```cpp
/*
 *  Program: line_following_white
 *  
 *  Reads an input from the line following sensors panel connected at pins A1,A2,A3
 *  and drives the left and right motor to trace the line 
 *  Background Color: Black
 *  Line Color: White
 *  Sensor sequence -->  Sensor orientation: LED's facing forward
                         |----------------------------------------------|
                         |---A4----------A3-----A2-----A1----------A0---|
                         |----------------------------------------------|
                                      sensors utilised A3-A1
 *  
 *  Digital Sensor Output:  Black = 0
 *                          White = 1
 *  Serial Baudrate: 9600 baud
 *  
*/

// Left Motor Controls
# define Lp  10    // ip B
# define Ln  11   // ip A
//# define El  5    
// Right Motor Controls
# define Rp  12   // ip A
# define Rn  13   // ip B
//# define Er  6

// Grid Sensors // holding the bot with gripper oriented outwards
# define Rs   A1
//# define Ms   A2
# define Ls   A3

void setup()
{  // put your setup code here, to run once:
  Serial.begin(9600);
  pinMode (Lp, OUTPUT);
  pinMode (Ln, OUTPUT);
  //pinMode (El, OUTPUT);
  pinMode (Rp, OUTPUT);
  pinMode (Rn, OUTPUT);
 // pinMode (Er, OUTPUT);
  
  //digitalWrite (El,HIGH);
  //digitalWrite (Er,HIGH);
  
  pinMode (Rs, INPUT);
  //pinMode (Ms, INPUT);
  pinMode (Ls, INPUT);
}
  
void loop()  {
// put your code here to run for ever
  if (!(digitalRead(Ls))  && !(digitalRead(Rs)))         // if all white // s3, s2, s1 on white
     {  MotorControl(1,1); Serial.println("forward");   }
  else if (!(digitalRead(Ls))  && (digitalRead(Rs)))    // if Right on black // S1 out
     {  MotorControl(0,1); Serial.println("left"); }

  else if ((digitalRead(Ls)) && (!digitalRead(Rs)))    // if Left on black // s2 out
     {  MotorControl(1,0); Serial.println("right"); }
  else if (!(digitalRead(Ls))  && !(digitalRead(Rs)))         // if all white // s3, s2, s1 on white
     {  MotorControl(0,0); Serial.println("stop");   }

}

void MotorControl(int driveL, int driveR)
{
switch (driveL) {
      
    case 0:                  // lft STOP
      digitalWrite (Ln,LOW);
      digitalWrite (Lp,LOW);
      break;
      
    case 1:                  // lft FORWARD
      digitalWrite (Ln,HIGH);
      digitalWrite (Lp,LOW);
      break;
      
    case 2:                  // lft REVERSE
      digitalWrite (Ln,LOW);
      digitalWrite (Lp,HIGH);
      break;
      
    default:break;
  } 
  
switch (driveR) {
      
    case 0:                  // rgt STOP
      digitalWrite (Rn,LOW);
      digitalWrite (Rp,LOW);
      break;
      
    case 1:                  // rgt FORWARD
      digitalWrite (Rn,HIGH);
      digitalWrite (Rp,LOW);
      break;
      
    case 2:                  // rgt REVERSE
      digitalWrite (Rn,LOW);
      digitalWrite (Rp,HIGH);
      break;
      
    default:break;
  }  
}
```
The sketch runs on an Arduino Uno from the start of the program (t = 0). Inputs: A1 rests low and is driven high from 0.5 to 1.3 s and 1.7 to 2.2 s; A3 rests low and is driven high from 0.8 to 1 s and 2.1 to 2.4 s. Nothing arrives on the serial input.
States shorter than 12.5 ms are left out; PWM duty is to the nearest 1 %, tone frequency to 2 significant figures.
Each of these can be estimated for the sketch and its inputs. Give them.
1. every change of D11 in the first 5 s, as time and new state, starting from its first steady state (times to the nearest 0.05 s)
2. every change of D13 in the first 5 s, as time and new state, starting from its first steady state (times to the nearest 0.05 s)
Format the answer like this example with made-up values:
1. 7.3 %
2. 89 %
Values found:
1. 0 s high; 0.5 s low; 1.3 s high; 1.7 s low; 2.2 s high
2. 0 s high; 2.2 s low; 2.4 s high
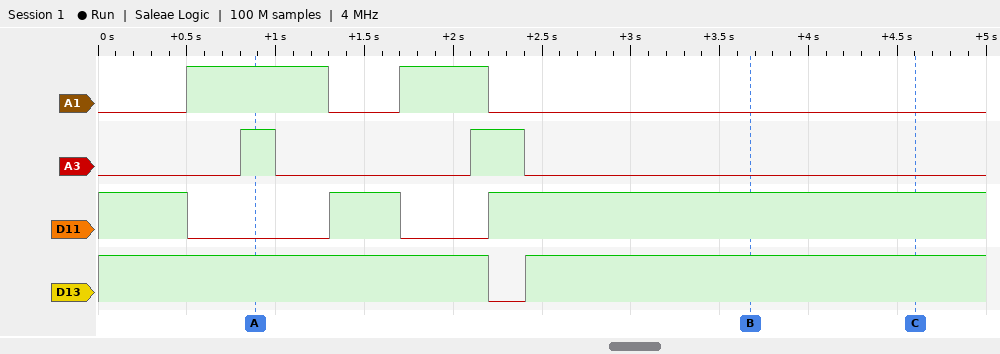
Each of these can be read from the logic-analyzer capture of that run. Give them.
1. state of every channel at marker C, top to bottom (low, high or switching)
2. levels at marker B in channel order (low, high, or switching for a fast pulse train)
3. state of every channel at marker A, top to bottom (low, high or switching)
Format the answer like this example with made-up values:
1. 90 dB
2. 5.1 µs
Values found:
1. A1 low, A3 low, D11 high, D13 high
2. A1 low, A3 low, D11 high, D13 high
3. A1 high, A3 high, D11 low, D13 high
